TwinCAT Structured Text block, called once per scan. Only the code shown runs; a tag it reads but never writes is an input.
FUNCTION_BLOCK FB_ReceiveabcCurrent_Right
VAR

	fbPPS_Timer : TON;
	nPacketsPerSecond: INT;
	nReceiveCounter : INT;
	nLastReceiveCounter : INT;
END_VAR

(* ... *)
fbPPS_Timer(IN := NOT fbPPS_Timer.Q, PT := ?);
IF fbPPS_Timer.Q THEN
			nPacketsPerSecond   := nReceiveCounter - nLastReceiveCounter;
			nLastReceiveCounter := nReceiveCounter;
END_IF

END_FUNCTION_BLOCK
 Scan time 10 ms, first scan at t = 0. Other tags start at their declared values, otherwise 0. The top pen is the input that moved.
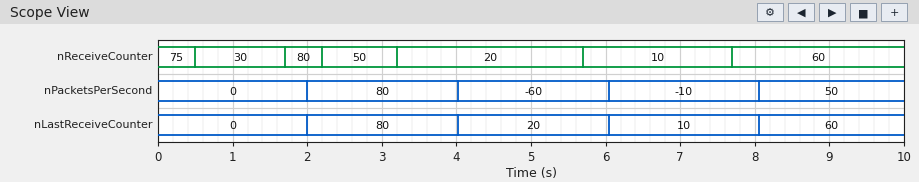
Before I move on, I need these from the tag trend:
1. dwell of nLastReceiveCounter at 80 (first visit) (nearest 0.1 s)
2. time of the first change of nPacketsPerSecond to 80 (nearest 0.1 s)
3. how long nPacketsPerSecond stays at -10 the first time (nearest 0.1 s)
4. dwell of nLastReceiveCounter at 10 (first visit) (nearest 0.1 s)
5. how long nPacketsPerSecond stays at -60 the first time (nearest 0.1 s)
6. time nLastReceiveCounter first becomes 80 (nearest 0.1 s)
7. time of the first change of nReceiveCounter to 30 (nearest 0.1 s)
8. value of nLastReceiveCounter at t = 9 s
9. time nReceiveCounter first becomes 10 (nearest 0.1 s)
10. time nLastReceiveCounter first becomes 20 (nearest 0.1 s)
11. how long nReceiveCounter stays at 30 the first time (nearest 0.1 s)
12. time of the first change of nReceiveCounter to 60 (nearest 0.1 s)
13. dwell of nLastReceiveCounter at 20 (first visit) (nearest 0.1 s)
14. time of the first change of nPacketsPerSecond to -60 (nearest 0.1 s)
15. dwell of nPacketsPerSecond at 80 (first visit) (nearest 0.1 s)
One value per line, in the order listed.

2.0 s
2.0 s
2.0 s
2.0 s
2.0 s
2.0 s
0.5 s
60
5.7 s
4.0 s
1.2 s
7.7 s
2.0 s
4.0 s
2.0 s
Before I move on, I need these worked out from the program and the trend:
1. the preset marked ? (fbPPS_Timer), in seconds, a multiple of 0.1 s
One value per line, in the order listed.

2.0 s
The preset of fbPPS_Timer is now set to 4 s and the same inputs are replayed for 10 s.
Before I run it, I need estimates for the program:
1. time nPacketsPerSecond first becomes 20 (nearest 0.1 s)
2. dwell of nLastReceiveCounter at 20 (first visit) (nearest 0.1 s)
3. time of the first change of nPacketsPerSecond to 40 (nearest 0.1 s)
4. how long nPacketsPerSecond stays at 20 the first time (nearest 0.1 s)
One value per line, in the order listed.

4.0 s
4.0 s
8.0 s
4.0 s
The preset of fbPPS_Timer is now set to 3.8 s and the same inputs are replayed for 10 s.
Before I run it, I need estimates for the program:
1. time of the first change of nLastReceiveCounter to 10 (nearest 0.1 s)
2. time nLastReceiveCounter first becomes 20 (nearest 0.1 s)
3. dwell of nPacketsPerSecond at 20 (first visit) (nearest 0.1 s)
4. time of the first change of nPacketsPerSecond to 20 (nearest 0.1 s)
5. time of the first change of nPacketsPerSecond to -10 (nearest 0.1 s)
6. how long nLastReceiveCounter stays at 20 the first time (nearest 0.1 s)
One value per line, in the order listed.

7.6 s
3.8 s
3.8 s
3.8 s
7.6 s
3.8 s
